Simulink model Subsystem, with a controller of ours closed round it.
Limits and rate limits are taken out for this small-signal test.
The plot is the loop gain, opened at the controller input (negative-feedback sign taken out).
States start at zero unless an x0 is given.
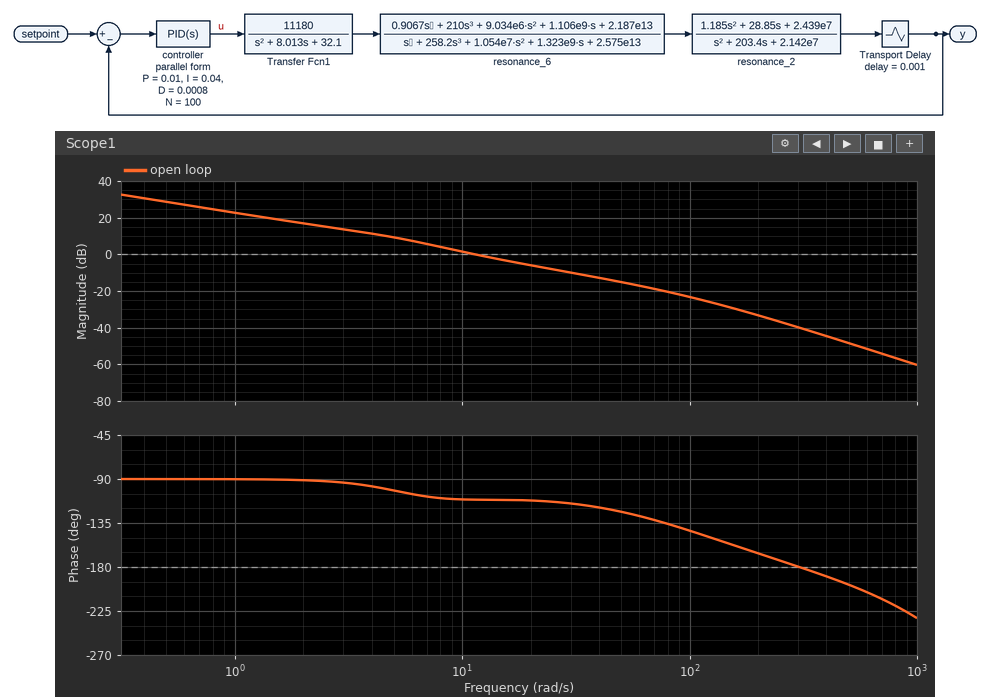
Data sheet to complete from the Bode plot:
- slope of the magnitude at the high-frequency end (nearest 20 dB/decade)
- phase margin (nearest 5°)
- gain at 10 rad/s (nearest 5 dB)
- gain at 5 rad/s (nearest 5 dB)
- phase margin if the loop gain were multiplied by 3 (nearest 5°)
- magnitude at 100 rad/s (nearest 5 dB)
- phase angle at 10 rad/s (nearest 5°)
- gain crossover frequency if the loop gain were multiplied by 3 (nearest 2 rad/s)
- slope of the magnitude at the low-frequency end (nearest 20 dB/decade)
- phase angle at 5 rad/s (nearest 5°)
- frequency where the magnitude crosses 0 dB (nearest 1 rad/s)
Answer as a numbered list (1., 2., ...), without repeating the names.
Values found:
1. -40 dB/decade
2. 70°
3. 0 dB
4. 10 dB
5. 65°
6. -25 dB
7. -110°
8. 28 rad/s
9. -20 dB/decade
10. -100°
11. 11 rad/s
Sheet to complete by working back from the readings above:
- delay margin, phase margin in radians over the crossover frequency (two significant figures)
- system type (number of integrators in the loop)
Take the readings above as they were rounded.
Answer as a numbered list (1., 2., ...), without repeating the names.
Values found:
1. 0.11 s
2. 1
